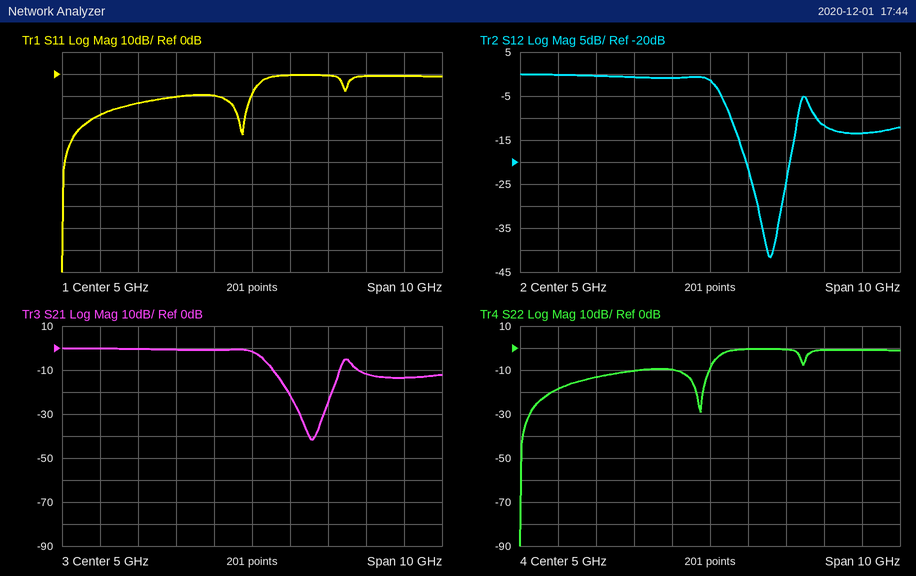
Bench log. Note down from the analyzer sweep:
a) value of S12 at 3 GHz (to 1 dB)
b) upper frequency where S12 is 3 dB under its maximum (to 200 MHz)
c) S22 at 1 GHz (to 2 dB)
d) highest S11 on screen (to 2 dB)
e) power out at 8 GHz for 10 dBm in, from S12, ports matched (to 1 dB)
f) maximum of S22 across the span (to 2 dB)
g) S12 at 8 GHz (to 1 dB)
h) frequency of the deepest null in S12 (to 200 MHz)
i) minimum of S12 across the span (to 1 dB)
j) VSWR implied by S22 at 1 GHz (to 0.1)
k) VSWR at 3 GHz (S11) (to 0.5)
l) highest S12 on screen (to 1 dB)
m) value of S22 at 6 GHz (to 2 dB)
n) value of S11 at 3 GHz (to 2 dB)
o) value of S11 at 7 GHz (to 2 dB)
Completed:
-1 dB
5.2 GHz
-18 dB
0 dB
-2 dBm
0 dB
-12 dB
6.6 GHz
-42 dB
1.3
2.0
0 dB
0 dB
-10 dB
0 dB
